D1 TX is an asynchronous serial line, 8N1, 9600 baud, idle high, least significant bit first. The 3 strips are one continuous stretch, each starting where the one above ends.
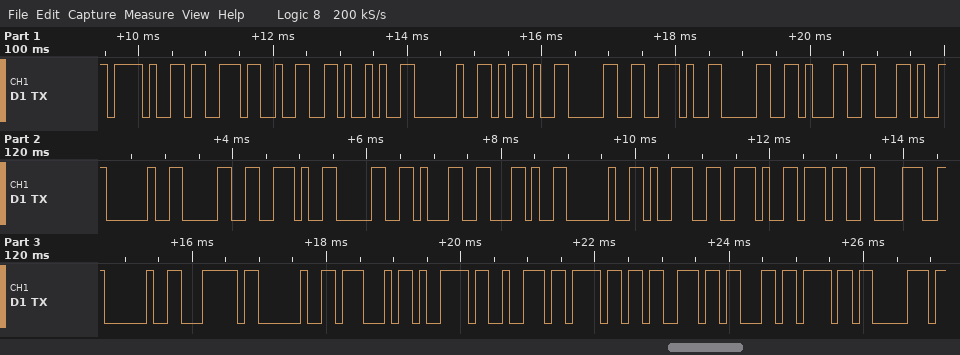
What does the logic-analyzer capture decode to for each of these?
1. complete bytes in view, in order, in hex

2F 73 32 29 20 2D 30 2E 30 31 2C 20 30 2E 30 31 2C 20 39 2E 37 38 20 7C 20 47 79 72 6F 73 63 6F 70
